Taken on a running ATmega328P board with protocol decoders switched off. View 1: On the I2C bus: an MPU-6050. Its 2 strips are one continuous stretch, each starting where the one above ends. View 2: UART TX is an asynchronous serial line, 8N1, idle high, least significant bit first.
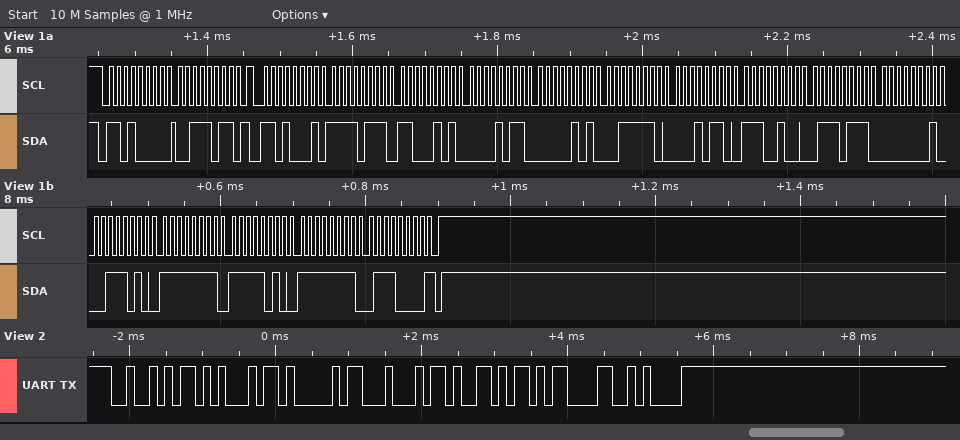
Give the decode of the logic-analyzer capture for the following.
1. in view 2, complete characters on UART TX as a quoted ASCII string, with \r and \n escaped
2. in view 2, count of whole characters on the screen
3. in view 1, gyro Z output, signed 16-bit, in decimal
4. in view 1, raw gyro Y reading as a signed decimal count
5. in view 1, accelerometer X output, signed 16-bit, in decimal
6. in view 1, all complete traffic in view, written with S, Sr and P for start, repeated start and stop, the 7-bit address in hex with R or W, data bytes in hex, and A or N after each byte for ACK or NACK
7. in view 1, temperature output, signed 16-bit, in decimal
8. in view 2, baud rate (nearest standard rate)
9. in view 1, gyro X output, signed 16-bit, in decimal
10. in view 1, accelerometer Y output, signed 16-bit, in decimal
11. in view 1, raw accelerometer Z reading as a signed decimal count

"READY\r\n"
7
-144
-6
-2107
S 68W A 3B A Sr 68R A F7 A C5 A 0B A 05 A 3E A 16 A E4 A 77 A 01 A 3A A FF A FA A FF A 70 N P
-7049
9600 baud
314
2821
15894
